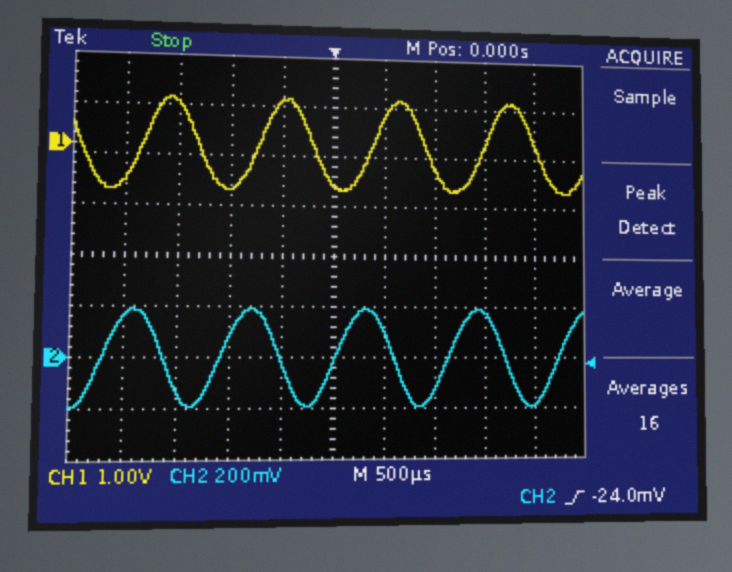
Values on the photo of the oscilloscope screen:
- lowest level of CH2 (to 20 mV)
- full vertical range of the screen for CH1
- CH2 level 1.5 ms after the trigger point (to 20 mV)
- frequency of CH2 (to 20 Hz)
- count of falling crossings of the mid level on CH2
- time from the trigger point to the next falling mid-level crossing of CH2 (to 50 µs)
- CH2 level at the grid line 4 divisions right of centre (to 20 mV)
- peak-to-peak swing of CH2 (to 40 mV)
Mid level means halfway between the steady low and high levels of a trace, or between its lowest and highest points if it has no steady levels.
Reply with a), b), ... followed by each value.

a) -200 mV
b) 8 V
c) 180 mV
d) 900 Hz
e) 4
f) 600 µs
g) -180 mV
h) 400 mV
